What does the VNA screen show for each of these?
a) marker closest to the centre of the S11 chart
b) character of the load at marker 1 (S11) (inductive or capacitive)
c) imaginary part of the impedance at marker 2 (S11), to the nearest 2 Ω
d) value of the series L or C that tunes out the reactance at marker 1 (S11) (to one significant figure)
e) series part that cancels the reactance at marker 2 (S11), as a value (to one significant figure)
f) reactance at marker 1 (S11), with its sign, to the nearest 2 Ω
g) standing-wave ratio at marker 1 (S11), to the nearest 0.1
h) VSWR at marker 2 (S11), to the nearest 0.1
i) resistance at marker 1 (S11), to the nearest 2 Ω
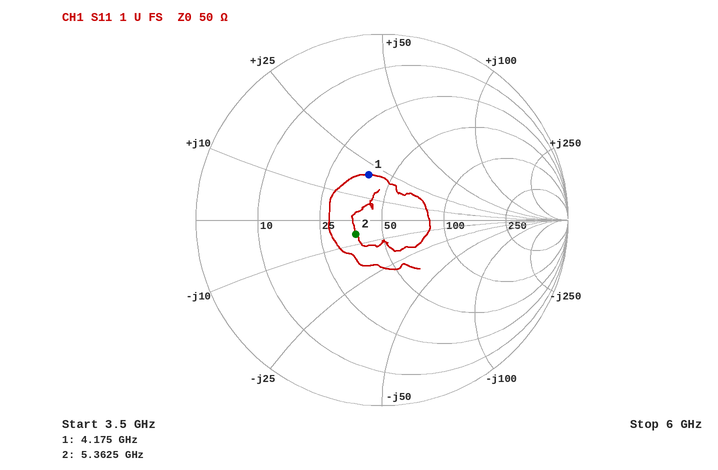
marker 2
inductive
-6 Ω
2 pF
200 pH
+20 Ω
1.7
1.4
38 Ω
